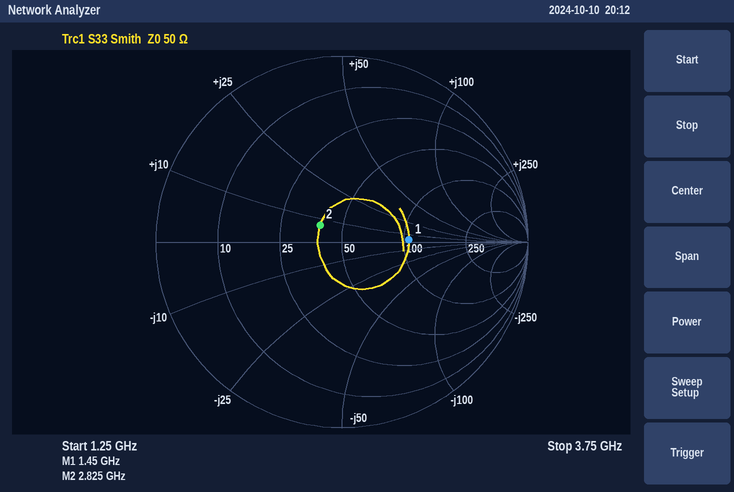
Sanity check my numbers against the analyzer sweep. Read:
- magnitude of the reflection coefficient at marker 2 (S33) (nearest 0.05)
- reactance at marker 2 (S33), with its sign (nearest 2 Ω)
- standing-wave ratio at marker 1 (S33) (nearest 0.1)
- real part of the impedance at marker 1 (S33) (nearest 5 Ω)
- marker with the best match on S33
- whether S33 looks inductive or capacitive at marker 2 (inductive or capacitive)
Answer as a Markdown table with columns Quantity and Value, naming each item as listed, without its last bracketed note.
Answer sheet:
| Quantity | Value |
|---|---|
| magnitude of the reflection coefficient at marker 2 (S33) | 0.15 |
| reactance at marker 2 (S33), with its sign | +8 Ω |
| standing-wave ratio at marker 1 (S33) | 2.1 |
| real part of the impedance at marker 1 (S33) | 105 Ω |
| marker with the best match on S33 | marker 2 |
| whether S33 looks inductive or capacitive at marker 2 | inductive |
